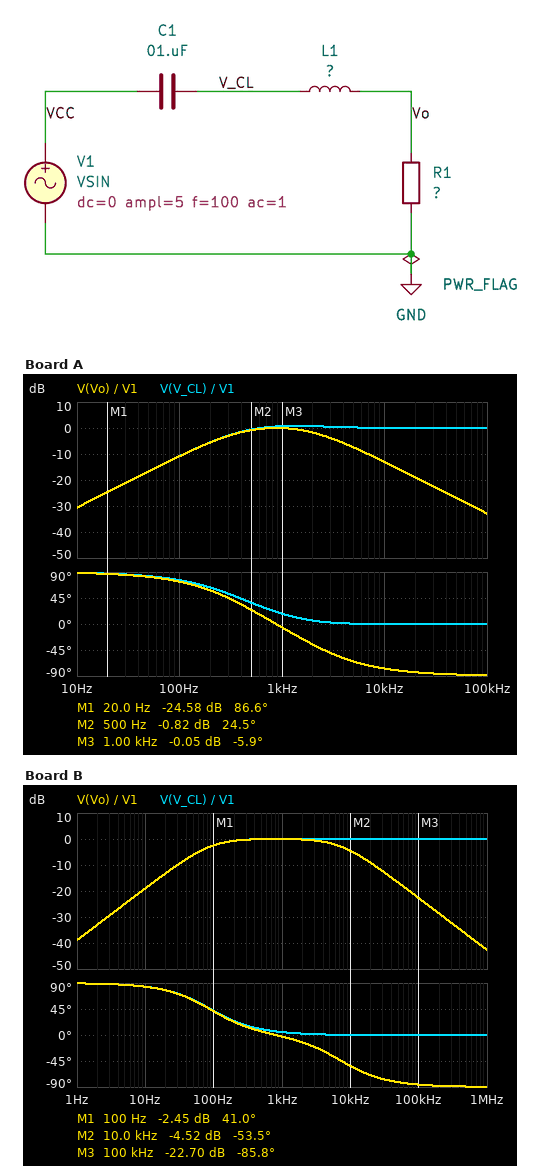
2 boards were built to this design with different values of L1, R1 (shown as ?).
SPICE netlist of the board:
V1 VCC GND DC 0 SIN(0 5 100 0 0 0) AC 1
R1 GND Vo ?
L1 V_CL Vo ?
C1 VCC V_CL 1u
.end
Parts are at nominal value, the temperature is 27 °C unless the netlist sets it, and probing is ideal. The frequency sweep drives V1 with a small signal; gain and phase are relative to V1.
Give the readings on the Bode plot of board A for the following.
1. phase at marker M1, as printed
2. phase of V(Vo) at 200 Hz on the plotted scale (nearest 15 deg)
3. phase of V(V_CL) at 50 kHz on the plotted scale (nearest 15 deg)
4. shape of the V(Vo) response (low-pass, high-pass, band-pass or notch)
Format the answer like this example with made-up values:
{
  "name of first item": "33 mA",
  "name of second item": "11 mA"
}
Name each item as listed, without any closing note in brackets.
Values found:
{
  "phase at marker M1, as printed": "86.6 deg",
  "phase of V(Vo) at 200 Hz on the plotted scale": "60 deg",
  "phase of V(V_CL) at 50 kHz on the plotted scale": "0 deg",
  "shape of the V(Vo) response": "band-pass"
}
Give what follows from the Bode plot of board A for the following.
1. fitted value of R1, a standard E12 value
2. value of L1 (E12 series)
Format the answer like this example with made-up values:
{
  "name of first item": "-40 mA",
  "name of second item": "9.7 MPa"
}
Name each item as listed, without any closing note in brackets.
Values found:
{
  "fitted value of R1, a standard E12 value": "470 Ω",
  "value of L1": "33 mH"
}
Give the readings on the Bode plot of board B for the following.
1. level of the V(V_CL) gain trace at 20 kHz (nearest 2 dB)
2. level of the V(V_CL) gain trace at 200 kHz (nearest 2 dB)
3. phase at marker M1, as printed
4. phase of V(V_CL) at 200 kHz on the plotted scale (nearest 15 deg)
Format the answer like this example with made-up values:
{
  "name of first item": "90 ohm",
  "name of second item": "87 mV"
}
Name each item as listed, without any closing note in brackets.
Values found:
{
  "level of the V(V_CL) gain trace at 20 kHz": "0 dB",
  "level of the V(V_CL) gain trace at 200 kHz": "0 dB",
  "phase at marker M1, as printed": "41.0 deg",
  "phase of V(V_CL) at 200 kHz on the plotted scale": "0 deg"
}
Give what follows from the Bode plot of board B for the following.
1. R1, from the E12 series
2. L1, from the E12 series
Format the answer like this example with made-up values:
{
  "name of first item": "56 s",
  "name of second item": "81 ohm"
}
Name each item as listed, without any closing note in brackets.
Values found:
{
  "R1, from the E12 series": "1.8 kΩ",
  "L1, from the E12 series": "39 mH"
}
